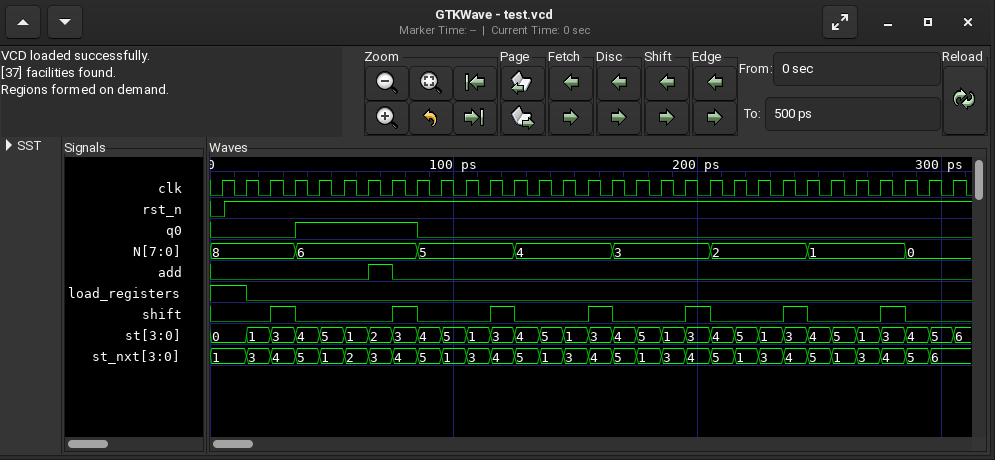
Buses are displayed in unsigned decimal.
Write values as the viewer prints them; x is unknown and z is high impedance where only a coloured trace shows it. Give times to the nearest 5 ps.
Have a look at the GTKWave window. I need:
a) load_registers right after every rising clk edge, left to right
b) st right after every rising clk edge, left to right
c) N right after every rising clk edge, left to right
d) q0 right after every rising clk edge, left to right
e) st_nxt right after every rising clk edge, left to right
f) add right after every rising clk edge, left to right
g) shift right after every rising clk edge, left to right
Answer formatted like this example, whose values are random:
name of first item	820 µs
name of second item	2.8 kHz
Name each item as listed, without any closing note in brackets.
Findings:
load_registers right after every rising clk edge, left to right	1 0 0 0 0 0 0 0 0 0 0 0 0 0 0 0 0 0 0 0 0 0 0 0 0 0 0 0 0 0 0
st right after every rising clk edge, left to right	0, 1, 3, 4, 5, 1, 2, 3, 4, 5, 1, 3, 4, 5, 1, 3, 4, 5, 1, 3, 4, 5, 1, 3, 4, 5, 1, 3, 4, 5, 6
N right after every rising clk edge, left to right	8, 8, 8, 6, 6, 6, 6, 6, 5, 5, 5, 5, 4, 4, 4, 4, 3, 3, 3, 3, 2, 2, 2, 2, 1, 1, 1, 1, 0, 0, 0
q0 right after every rising clk edge, left to right	0 0 0 1 1 1 1 1 0 0 0 0 0 0 0 0 0 0 0 0 0 0 0 0 0 0 0 0 0 0 0
st_nxt right after every rising clk edge, left to right	1, 3, 4, 5, 1, 2, 3, 4, 5, 1, 3, 4, 5, 1, 3, 4, 5, 1, 3, 4, 5, 1, 3, 4, 5, 1, 3, 4, 5, 6, 6
add right after every rising clk edge, left to right	0 0 0 0 0 0 1 0 0 0 0 0 0 0 0 0 0 0 0 0 0 0 0 0 0 0 0 0 0 0 0
shift right after every rising clk edge, left to right	0 0 1 0 0 0 0 1 0 0 0 1 0 0 0 1 0 0 0 1 0 0 0 1 0 0 0 1 0 0 0
